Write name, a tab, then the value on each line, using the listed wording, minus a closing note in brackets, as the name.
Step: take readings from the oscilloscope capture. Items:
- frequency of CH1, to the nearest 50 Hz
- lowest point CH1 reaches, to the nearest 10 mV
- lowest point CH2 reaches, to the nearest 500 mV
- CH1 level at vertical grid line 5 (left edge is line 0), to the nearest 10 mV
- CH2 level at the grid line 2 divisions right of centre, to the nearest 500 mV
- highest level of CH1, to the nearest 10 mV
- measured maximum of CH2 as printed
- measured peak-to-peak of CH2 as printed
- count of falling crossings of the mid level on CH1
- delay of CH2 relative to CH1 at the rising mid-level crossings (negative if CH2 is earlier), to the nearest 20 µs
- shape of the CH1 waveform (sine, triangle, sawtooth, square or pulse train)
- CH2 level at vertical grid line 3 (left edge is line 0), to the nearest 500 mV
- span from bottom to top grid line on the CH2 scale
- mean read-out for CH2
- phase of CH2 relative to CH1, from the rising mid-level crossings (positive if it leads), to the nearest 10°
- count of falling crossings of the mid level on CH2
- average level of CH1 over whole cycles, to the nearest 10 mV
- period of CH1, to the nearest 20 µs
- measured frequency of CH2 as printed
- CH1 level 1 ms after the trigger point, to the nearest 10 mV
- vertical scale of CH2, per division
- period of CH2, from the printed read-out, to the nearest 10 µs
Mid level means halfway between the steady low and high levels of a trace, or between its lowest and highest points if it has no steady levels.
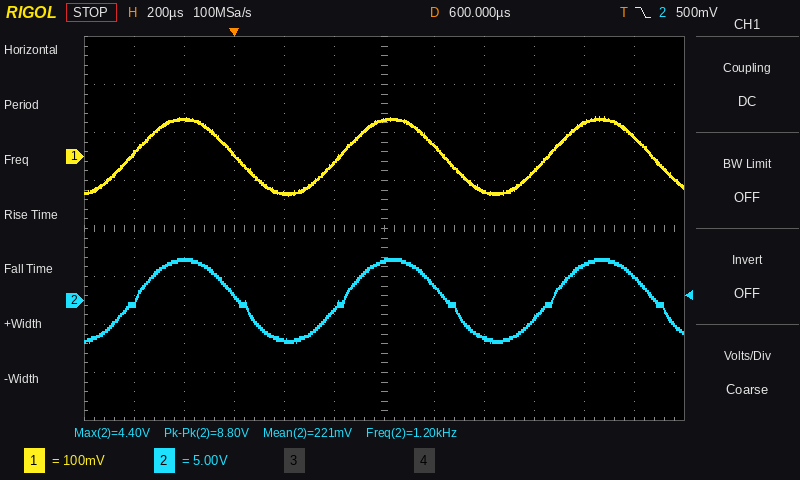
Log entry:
frequency of CH1, to the nearest 50 Hz	1.20 kHz
lowest point CH1 reaches, to the nearest 10 mV	-80 mV
lowest point CH2 reaches, to the nearest 500 mV	-4.5 V
CH1 level at vertical grid line 5 (left edge is line 0), to the nearest 10 mV	-10 mV
CH2 level at the grid line 2 divisions right of centre, to the nearest 500 mV	-4.0 V
highest level of CH1, to the nearest 10 mV	80 mV
measured maximum of CH2 as printed	4.40 V
measured peak-to-peak of CH2 as printed	8.80 V
count of falling crossings of the mid level on CH1	3
delay of CH2 relative to CH1 at the rising mid-level crossings (negative if CH2 is earlier), to the nearest 20 µs	+20 µs
shape of the CH1 waveform	sine
CH2 level at vertical grid line 3 (left edge is line 0), to the nearest 500 mV	500 mV
span from bottom to top grid line on the CH2 scale	40 V
mean read-out for CH2	221 mV
phase of CH2 relative to CH1, from the rising mid-level crossings (positive if it leads), to the nearest 10°	-10°
count of falling crossings of the mid level on CH2	3
average level of CH1 over whole cycles, to the nearest 10 mV	0 mV
period of CH1, to the nearest 20 µs	840 µs
measured frequency of CH2 as printed	1.20 kHz
CH1 level 1 ms after the trigger point, to the nearest 10 mV	-70 mV
vertical scale of CH2, per division	5 V
period of CH2, from the printed read-out, to the nearest 10 µs	830 µs
